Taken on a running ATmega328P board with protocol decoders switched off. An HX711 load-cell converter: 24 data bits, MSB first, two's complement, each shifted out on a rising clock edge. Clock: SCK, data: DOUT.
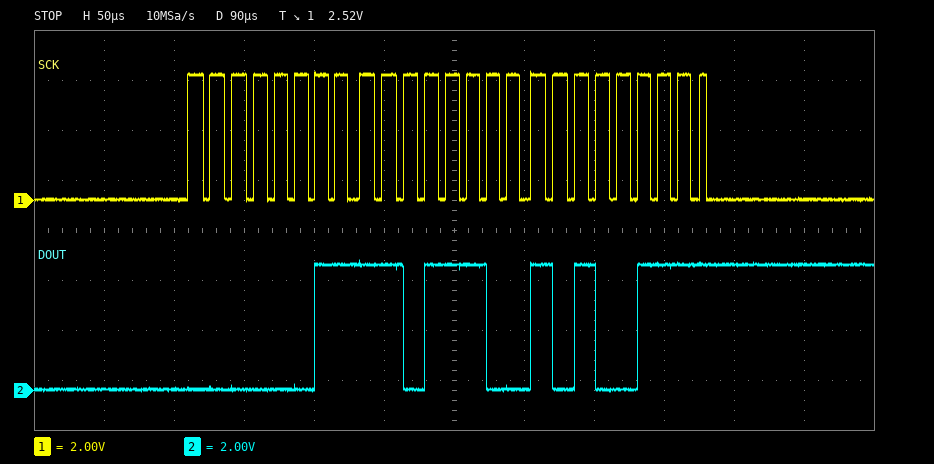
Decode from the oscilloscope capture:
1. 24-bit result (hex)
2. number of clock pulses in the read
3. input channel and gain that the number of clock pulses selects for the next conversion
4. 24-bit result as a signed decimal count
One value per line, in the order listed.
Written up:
0x03DCA7
25
channel A, gain 128
253095
